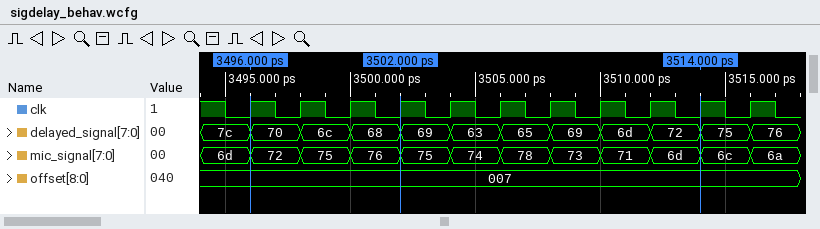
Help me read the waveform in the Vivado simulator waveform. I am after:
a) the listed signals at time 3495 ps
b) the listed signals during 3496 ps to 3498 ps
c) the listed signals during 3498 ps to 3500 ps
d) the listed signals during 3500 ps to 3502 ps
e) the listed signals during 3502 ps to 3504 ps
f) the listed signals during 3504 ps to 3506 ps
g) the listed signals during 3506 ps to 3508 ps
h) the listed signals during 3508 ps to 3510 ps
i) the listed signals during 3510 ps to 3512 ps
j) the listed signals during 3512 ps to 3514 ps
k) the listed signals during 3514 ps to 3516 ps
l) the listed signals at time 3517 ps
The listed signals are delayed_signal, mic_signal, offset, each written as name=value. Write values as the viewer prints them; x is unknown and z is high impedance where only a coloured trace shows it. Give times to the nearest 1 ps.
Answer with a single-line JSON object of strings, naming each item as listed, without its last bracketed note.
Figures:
{"the listed signals at time 3495 ps": "delayed_signal=7c, mic_signal=6d, offset=007", "the listed signals during 3496 ps to 3498 ps": "delayed_signal=70, mic_signal=72, offset=007", "the listed signals during 3498 ps to 3500 ps": "delayed_signal=6c, mic_signal=75, offset=007", "the listed signals during 3500 ps to 3502 ps": "delayed_signal=68, mic_signal=76, offset=007", "the listed signals during 3502 ps to 3504 ps": "delayed_signal=69, mic_signal=75, offset=007", "the listed signals during 3504 ps to 3506 ps": "delayed_signal=63, mic_signal=74, offset=007", "the listed signals during 3506 ps to 3508 ps": "delayed_signal=65, mic_signal=78, offset=007", "the listed signals during 3508 ps to 3510 ps": "delayed_signal=69, mic_signal=73, offset=007", "the listed signals during 3510 ps to 3512 ps": "delayed_signal=6d, mic_signal=71, offset=007", "the listed signals during 3512 ps to 3514 ps": "delayed_signal=72, mic_signal=6d, offset=007", "the listed signals during 3514 ps to 3516 ps": "delayed_signal=75, mic_signal=6c, offset=007", "the listed signals at time 3517 ps": "delayed_signal=76, mic_signal=6a, offset=007"}
